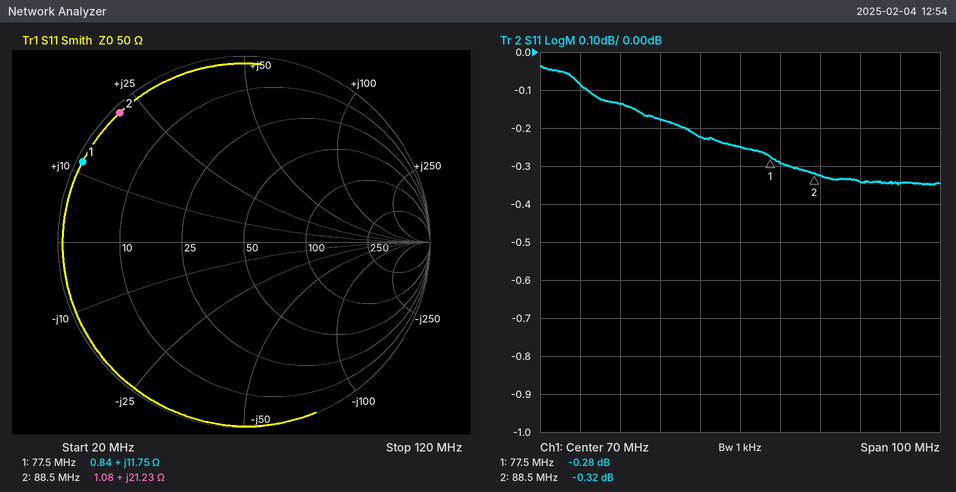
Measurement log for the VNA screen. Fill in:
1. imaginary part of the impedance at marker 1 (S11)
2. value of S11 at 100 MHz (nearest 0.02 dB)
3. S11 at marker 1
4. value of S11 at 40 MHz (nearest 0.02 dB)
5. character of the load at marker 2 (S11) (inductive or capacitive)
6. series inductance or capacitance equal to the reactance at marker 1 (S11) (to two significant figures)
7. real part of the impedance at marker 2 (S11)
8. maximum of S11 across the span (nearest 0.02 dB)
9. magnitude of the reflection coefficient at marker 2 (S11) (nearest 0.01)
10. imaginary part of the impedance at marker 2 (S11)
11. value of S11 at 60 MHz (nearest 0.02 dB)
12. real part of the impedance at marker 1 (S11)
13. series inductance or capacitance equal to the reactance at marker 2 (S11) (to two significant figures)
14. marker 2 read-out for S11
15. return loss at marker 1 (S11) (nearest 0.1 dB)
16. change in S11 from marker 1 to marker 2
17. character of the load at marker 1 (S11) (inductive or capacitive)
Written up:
+11.75 Ω
-0.34 dB
-0.28 dB
-0.14 dB
inductive
24 nH
1.08 Ω
-0.04 dB
0.96
+21.23 Ω
-0.22 dB
0.84 Ω
38 nH
-0.32 dB
0.3 dB
-0.04 dB
inductive
